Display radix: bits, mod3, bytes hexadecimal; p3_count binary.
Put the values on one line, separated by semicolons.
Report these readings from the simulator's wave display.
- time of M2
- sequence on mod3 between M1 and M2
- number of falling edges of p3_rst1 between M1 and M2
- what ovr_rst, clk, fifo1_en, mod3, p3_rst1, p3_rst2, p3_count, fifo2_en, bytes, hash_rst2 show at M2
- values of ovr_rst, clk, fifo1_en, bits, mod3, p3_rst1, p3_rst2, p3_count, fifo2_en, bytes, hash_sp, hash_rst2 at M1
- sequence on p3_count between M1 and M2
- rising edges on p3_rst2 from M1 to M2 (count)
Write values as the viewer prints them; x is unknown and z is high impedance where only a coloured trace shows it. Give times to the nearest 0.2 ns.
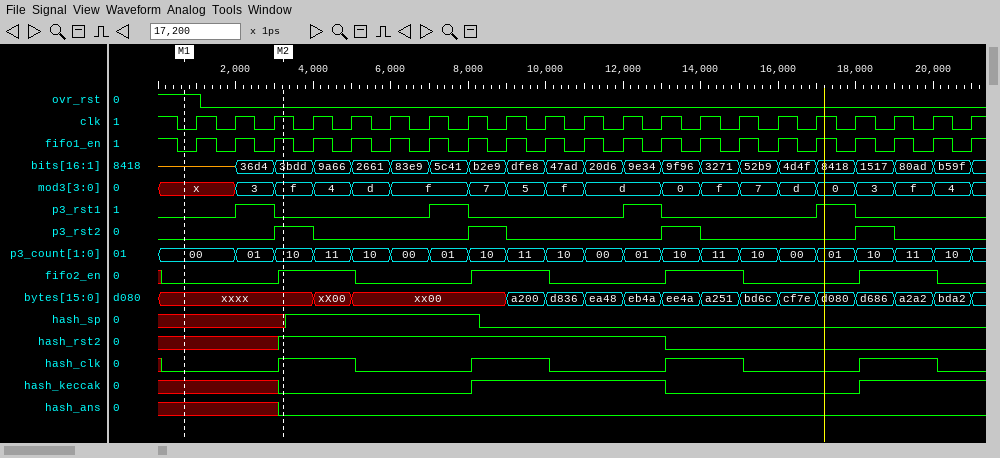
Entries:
3.2 ns; x, 3, f; 1; ovr_rst=0, clk=1, fifo1_en=1, mod3=f, p3_rst1=0, p3_rst2=1, p3_count=10, fifo2_en=1, bytes=xxxx, hash_rst2=1; ovr_rst=1, clk=0, fifo1_en=0, bits=z, mod3=x, p3_rst1=0, p3_rst2=0, p3_count=00, fifo2_en=0, bytes=xxxx, hash_sp=x, hash_rst2=x; 00, 01, 10; 1
